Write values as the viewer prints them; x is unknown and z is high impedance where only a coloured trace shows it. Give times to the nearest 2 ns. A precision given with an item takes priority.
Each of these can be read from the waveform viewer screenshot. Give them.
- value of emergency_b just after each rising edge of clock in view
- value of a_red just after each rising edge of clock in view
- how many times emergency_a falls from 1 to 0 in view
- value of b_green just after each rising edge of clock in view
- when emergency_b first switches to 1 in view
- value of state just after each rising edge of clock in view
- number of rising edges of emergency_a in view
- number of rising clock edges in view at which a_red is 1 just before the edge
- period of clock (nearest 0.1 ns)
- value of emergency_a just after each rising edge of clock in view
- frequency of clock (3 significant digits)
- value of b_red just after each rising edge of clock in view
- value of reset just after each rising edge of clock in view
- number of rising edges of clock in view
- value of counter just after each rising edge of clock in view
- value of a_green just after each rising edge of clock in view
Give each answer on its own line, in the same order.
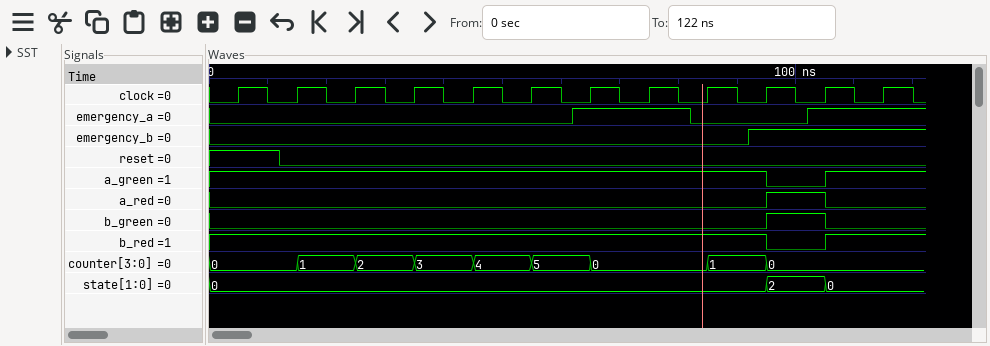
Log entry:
0 0 0 0 0 0 0 0 0 1 1 1
0 0 0 0 0 0 0 0 0 1 0 0
1
0 0 0 0 0 0 0 0 0 1 0 0
92 ns
0, 0, 0, 0, 0, 0, 0, 0, 0, 2, 0, 0
2
1
10 ns
0 0 0 0 0 0 1 1 0 0 1 1
100 MHz
1 1 1 1 1 1 1 1 1 0 1 1
1 0 0 0 0 0 0 0 0 0 0 0
12
0, 1, 2, 3, 4, 5, 0, 0, 1, 0, 0, 0
1 1 1 1 1 1 1 1 1 0 1 1
